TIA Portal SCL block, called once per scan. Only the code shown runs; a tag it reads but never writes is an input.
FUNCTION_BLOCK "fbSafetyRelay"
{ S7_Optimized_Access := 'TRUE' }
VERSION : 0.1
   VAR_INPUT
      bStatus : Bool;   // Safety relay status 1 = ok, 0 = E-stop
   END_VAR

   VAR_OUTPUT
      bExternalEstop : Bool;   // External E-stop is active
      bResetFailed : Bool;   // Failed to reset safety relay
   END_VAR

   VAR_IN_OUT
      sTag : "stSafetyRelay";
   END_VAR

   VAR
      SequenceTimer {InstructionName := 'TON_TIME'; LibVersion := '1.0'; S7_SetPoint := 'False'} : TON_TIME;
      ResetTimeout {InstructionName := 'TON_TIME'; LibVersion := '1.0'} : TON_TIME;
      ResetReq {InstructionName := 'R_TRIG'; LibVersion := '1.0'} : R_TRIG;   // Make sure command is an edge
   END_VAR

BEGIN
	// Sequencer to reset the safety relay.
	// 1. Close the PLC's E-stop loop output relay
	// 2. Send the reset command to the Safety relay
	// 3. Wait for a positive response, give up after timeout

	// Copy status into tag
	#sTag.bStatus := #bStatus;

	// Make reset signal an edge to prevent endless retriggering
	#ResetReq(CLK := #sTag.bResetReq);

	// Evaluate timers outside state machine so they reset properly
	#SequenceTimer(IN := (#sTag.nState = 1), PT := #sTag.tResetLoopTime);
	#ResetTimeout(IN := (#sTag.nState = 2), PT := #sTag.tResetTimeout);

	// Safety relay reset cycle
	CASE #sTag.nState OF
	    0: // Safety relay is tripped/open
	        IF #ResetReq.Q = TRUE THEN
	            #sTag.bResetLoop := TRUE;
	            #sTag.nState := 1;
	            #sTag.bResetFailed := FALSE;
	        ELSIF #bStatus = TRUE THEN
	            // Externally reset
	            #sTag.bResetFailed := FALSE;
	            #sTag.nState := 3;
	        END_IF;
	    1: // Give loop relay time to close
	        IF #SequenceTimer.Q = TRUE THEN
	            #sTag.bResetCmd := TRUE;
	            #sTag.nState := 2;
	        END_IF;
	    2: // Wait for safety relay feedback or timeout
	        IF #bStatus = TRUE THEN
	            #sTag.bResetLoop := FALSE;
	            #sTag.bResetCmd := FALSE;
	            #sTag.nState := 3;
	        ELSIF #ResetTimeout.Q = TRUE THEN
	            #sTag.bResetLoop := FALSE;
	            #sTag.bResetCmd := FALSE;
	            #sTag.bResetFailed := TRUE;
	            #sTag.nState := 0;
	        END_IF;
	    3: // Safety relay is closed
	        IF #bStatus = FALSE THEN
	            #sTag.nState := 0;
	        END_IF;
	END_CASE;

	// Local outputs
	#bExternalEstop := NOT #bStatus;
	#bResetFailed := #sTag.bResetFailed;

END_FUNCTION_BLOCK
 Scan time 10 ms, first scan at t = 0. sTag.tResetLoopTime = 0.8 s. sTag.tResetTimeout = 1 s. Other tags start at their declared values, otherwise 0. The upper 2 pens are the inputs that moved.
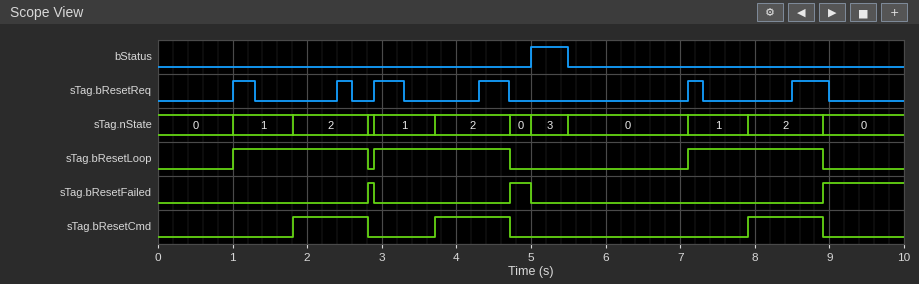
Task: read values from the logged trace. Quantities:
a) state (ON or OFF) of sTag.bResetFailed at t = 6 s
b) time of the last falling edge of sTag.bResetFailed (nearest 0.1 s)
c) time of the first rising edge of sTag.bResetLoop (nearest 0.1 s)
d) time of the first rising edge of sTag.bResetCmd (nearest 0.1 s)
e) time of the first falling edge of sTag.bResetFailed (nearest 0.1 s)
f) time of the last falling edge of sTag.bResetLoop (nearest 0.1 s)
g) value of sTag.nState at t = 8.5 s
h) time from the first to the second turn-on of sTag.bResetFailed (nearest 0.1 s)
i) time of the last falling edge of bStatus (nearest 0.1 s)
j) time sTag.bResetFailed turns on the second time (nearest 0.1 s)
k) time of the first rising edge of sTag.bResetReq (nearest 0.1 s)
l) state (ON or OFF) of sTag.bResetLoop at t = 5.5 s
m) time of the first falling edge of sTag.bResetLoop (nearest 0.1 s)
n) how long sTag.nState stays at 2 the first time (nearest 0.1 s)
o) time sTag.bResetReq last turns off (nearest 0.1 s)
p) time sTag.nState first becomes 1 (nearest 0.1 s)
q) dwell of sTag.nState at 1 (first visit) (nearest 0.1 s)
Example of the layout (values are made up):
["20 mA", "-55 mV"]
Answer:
["OFF", "5.0 s", "1.0 s", "1.8 s", "2.9 s", "8.9 s", "2", "1.9 s", "5.5 s", "4.7 s", "1.0 s", "OFF", "2.8 s", "1.0 s", "9.0 s", "1.0 s", "0.8 s"]
